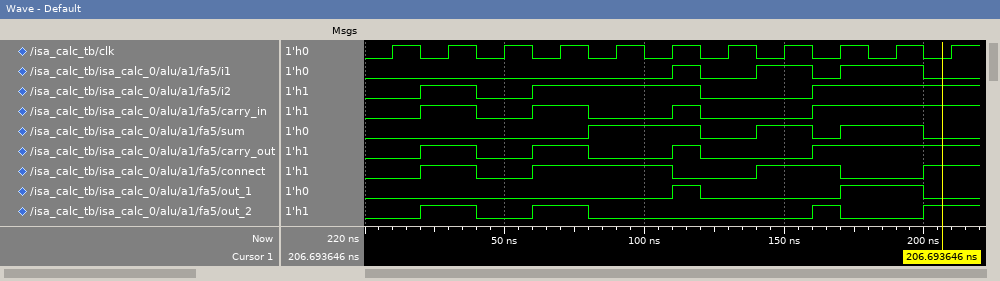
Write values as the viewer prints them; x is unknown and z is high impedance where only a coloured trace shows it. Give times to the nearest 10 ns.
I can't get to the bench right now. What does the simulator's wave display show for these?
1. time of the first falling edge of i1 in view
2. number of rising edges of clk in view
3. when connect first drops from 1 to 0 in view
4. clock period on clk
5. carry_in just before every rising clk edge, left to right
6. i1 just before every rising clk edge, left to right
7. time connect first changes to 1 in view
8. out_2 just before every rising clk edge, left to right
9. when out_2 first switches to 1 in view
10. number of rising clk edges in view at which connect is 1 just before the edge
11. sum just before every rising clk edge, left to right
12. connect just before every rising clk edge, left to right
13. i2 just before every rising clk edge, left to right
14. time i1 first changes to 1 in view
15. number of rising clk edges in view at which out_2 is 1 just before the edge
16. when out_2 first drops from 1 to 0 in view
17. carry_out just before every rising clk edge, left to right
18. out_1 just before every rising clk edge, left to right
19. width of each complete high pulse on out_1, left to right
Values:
120 ns
11
40 ns
20 ns
0 1 0 1 0 0 0 0 1 1 1
0 0 0 0 0 0 0 1 0 1 0
20 ns
0 1 0 1 0 0 0 0 1 0 1
20 ns
7
0 0 0 0 1 1 0 1 0 1 0
0 1 0 1 1 1 0 1 1 0 1
0 1 0 1 1 1 0 0 1 1 1
110 ns
4
40 ns
0 1 0 1 0 0 0 0 1 1 1
0 0 0 0 0 0 0 0 0 1 0
10 ns, 30 ns
